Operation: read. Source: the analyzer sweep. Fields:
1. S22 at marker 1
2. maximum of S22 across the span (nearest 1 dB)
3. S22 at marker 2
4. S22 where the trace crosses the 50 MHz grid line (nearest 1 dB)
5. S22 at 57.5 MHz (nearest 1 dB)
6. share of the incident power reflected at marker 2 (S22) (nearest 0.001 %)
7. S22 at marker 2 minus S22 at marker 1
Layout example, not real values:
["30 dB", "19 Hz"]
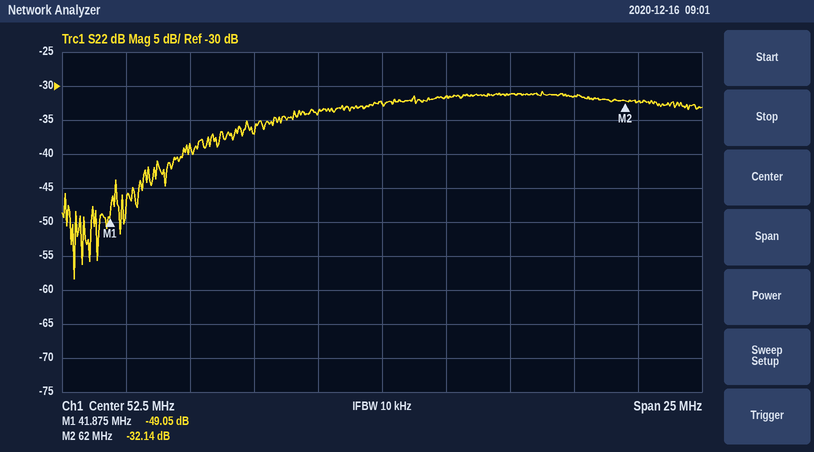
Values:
["-49.05 dB", "-31 dB", "-32.14 dB", "-34 dB", "-31 dB", "0.061 %", "16.91 dB"]
